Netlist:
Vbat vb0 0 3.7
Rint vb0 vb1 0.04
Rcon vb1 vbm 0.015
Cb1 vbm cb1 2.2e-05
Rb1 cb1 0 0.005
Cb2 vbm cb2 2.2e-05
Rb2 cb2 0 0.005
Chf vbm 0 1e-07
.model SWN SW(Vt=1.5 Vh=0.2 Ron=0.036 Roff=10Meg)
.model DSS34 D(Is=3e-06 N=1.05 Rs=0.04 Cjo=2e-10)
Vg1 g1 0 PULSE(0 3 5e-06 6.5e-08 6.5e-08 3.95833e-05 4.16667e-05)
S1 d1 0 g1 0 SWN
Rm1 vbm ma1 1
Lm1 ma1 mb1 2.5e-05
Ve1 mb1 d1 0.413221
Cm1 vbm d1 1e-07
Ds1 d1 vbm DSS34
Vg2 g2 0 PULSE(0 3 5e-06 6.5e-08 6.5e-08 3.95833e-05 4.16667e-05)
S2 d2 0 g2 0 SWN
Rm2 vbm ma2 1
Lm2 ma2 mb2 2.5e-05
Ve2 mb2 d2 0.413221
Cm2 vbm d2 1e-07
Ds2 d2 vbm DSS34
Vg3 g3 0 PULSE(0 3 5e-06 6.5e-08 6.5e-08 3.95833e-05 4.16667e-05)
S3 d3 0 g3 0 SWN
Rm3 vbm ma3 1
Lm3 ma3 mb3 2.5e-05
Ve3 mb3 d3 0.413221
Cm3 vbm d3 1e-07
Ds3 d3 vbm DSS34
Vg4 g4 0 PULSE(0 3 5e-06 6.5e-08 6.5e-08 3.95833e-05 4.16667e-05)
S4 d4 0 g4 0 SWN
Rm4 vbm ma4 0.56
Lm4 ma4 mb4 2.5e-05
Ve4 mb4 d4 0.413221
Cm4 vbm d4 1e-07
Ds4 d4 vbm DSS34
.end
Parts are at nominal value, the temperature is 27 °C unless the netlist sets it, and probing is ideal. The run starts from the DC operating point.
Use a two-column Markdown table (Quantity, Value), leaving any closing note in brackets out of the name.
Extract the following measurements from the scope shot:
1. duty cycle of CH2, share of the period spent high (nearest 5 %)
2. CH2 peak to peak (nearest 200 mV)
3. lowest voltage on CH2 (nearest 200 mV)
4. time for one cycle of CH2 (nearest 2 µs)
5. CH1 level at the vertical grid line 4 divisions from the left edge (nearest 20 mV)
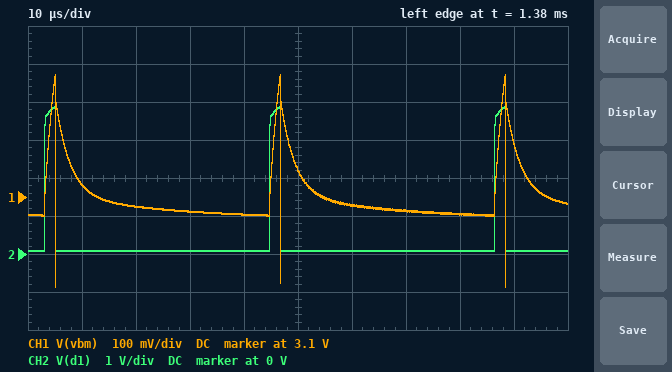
| Quantity | Value |
|---|---|
| duty cycle of CH2, share of the period spent high | 5 % |
| CH2 peak to peak | 3.8 V |
| lowest voltage on CH2 | 0 V |
| time for one cycle of CH2 | 42 µs |
| CH1 level at the vertical grid line 4 divisions from the left edge | 3.06 V |
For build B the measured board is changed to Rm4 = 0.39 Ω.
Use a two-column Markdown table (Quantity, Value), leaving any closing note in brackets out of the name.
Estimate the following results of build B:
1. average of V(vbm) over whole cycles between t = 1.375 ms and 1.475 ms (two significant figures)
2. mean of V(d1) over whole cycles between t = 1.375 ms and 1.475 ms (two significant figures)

| Quantity | Value |
|---|---|
| average of V(vbm) over whole cycles between t = 1.375 ms and 1.475 ms | 3.0 V |
| mean of V(d1) over whole cycles between t = 1.375 ms and 1.475 ms | 250 mV |
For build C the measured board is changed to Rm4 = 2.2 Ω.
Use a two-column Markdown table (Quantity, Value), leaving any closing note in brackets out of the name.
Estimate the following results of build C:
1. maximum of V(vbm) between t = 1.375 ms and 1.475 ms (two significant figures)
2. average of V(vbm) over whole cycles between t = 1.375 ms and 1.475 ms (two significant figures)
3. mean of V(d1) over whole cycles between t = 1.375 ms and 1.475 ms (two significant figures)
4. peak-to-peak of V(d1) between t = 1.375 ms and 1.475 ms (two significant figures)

| Quantity | Value |
|---|---|
| maximum of V(vbm) between t = 1.375 ms and 1.475 ms | 3.5 V |
| average of V(vbm) over whole cycles between t = 1.375 ms and 1.475 ms | 3.2 V |
| mean of V(d1) over whole cycles between t = 1.375 ms and 1.475 ms | 270 mV |
| peak-to-peak of V(d1) between t = 1.375 ms and 1.475 ms | 3.9 V |
